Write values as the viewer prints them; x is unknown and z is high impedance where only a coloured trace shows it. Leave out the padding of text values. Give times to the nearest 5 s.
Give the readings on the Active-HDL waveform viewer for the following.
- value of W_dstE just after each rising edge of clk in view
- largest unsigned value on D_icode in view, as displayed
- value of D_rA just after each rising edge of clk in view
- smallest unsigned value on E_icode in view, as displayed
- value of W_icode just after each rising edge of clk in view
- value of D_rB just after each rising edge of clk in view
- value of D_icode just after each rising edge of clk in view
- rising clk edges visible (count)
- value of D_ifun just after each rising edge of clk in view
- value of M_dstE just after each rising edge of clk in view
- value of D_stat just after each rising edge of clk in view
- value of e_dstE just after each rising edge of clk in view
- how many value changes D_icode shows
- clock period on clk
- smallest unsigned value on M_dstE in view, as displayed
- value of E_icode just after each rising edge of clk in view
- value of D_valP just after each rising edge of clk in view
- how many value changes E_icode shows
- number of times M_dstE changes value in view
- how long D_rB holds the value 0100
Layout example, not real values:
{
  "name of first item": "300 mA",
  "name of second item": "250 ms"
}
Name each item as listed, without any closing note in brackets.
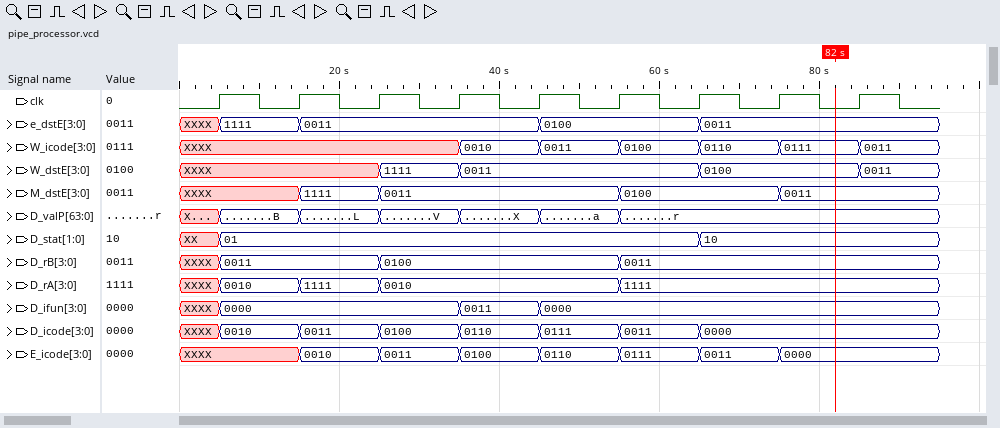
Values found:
{
  "value of W_dstE just after each rising edge of clk in view": "XXXX, XXXX, 1111, 0011, 0011, 0011, 0100, 0100, 0011",
  "largest unsigned value on D_icode in view, as displayed": "0111",
  "value of D_rA just after each rising edge of clk in view": "0010, 1111, 0010, 0010, 0010, 1111, 1111, 1111, 1111",
  "smallest unsigned value on E_icode in view, as displayed": "0000",
  "value of W_icode just after each rising edge of clk in view": "XXXX, XXXX, XXXX, 0010, 0011, 0100, 0110, 0111, 0011",
  "value of D_rB just after each rising edge of clk in view": "0011, 0011, 0100, 0100, 0100, 0011, 0011, 0011, 0011",
  "value of D_icode just after each rising edge of clk in view": "0010, 0011, 0100, 0110, 0111, 0011, 0000, 0000, 0000",
  "rising clk edges visible": "9",
  "value of D_ifun just after each rising edge of clk in view": "0000, 0000, 0000, 0011, 0000, 0000, 0000, 0000, 0000",
  "value of M_dstE just after each rising edge of clk in view": "XXXX, 1111, 0011, 0011, 0011, 0100, 0100, 0011, 0011",
  "value of D_stat just after each rising edge of clk in view": "01, 01, 01, 01, 01, 01, 10, 10, 10",
  "value of e_dstE just after each rising edge of clk in view": "1111, 0011, 0011, 0011, 0100, 0100, 0011, 0011, 0011",
  "how many value changes D_icode shows": "7",
  "clock period on clk": "10 s",
  "smallest unsigned value on M_dstE in view, as displayed": "0011",
  "value of E_icode just after each rising edge of clk in view": "XXXX, 0010, 0011, 0100, 0110, 0111, 0011, 0000, 0000",
  "value of D_valP just after each rising edge of clk in view": "B, L, V, X, a, r, r, r, r",
  "how many value changes E_icode shows": "7",
  "number of times M_dstE changes value in view": "4",
  "how long D_rB holds the value 0100": "30 s"
}
